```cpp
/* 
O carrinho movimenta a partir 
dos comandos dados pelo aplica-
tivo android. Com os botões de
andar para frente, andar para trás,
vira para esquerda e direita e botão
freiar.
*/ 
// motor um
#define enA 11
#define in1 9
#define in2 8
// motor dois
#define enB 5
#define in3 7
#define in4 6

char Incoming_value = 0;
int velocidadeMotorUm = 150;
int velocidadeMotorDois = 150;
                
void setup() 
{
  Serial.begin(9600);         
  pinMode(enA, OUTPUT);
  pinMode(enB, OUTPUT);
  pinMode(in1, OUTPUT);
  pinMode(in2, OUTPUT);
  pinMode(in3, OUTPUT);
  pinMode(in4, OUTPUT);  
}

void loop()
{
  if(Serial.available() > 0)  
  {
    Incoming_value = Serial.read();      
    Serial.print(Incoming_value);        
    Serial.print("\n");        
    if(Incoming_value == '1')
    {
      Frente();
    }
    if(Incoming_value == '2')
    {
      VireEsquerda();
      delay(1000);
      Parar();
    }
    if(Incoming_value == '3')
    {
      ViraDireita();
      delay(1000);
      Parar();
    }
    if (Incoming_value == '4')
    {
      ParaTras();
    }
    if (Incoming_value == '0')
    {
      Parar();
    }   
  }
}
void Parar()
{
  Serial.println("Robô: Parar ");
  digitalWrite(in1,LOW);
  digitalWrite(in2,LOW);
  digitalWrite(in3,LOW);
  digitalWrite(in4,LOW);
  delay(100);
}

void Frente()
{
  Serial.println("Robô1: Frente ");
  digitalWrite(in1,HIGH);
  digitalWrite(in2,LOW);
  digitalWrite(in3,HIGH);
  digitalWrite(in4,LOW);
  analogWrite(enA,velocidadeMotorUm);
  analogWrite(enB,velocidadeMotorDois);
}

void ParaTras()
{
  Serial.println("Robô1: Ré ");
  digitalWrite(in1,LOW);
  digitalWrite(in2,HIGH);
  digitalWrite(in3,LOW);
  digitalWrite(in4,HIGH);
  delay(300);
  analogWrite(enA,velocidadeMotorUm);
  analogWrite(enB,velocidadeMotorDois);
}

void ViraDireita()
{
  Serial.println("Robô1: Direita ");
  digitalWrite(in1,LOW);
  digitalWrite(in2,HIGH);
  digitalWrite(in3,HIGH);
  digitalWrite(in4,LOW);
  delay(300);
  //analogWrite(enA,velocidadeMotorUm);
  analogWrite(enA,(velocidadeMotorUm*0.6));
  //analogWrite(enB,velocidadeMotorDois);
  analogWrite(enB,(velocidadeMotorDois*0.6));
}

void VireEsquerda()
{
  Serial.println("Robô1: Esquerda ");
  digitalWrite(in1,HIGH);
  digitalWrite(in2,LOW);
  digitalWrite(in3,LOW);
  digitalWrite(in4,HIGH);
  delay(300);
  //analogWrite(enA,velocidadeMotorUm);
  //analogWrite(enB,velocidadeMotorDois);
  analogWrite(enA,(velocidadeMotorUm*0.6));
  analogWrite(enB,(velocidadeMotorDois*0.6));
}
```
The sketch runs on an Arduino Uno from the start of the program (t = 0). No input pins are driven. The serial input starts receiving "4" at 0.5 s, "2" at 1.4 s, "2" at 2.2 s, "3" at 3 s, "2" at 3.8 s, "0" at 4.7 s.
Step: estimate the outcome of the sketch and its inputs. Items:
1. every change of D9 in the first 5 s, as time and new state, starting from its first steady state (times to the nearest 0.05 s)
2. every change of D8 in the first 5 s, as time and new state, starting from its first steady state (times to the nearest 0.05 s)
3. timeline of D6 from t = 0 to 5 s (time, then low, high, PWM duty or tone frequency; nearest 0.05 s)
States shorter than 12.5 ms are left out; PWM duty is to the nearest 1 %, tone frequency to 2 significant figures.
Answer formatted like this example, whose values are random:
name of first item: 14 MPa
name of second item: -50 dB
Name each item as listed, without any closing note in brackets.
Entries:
every change of D9 in the first 5 s, as time and new state, starting from its first steady state: 0 s low; 1.4 s high; 2.7 s low; 2.8 s high; 4.1 s low
every change of D8 in the first 5 s, as time and new state, starting from its first steady state: 0 s low; 0.5 s high; 1.4 s low; 4.2 s high
timeline of D6 from t = 0 to 5 s: 0 s low; 0.5 s high; 2.7 s low; 2.8 s high; 4.1 s low
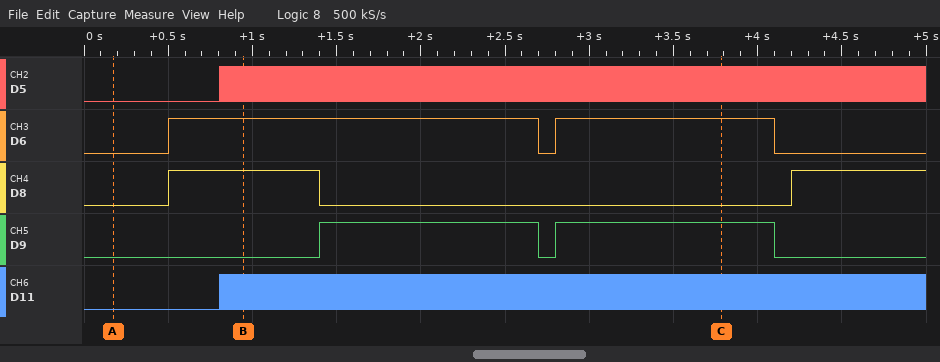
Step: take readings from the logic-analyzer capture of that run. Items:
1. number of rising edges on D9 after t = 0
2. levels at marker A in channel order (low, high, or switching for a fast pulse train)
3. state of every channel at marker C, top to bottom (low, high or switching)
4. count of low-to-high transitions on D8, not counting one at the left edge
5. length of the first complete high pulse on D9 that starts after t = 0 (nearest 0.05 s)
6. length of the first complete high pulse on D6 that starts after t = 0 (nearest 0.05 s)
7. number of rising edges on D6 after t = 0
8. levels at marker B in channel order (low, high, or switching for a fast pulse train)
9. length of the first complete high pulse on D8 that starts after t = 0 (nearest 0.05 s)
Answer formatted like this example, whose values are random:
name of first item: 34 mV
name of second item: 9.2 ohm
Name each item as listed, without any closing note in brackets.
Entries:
number of rising edges on D9 after t = 0: 2
levels at marker A in channel order: D5 low, D6 low, D8 low, D9 low, D11 low
state of every channel at marker C, top to bottom: D5 switching, D6 high, D8 low, D9 high, D11 switching
count of low-to-high transitions on D8, not counting one at the left edge: 2
length of the first complete high pulse on D9 that starts after t = 0: 1.30 s
length of the first complete high pulse on D6 that starts after t = 0: 2.20 s
number of rising edges on D6 after t = 0: 2
levels at marker B in channel order: D5 switching, D6 high, D8 high, D9 low, D11 switching
length of the first complete high pulse on D8 that starts after t = 0: 0.90 s
